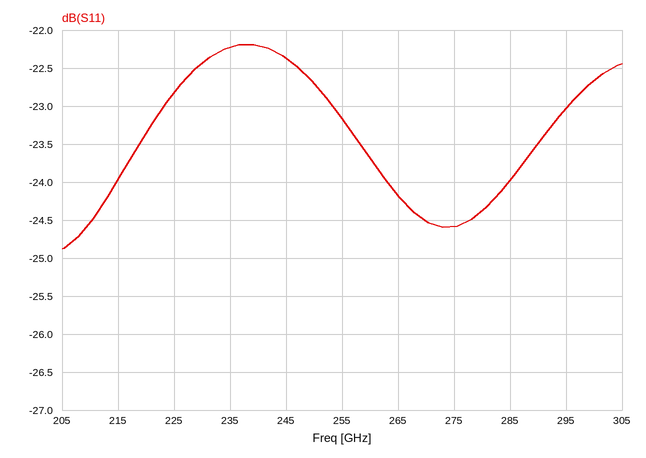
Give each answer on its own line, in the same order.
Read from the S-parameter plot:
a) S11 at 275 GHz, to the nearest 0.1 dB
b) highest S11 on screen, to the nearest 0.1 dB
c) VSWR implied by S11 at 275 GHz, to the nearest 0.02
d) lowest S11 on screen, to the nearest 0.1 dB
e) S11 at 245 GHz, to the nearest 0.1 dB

-24.6 dB
-22.2 dB
1.12
-24.9 dB
-22.4 dB
